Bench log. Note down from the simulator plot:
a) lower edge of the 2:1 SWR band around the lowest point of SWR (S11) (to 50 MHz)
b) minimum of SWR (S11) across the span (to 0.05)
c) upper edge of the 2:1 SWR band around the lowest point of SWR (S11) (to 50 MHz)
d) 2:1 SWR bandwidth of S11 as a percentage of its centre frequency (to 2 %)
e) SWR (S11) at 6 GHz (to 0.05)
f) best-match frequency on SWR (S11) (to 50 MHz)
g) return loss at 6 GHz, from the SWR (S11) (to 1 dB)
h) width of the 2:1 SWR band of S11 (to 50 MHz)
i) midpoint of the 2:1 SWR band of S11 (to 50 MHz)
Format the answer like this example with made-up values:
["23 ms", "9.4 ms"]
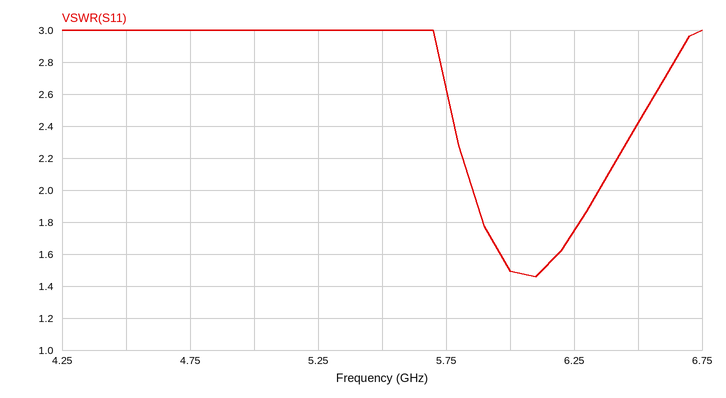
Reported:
["5.85 GHz", "1.45", "6.35 GHz", "8 %", "1.50", "6.10 GHz", "14 dB", "500 MHz", "6.10 GHz"]
